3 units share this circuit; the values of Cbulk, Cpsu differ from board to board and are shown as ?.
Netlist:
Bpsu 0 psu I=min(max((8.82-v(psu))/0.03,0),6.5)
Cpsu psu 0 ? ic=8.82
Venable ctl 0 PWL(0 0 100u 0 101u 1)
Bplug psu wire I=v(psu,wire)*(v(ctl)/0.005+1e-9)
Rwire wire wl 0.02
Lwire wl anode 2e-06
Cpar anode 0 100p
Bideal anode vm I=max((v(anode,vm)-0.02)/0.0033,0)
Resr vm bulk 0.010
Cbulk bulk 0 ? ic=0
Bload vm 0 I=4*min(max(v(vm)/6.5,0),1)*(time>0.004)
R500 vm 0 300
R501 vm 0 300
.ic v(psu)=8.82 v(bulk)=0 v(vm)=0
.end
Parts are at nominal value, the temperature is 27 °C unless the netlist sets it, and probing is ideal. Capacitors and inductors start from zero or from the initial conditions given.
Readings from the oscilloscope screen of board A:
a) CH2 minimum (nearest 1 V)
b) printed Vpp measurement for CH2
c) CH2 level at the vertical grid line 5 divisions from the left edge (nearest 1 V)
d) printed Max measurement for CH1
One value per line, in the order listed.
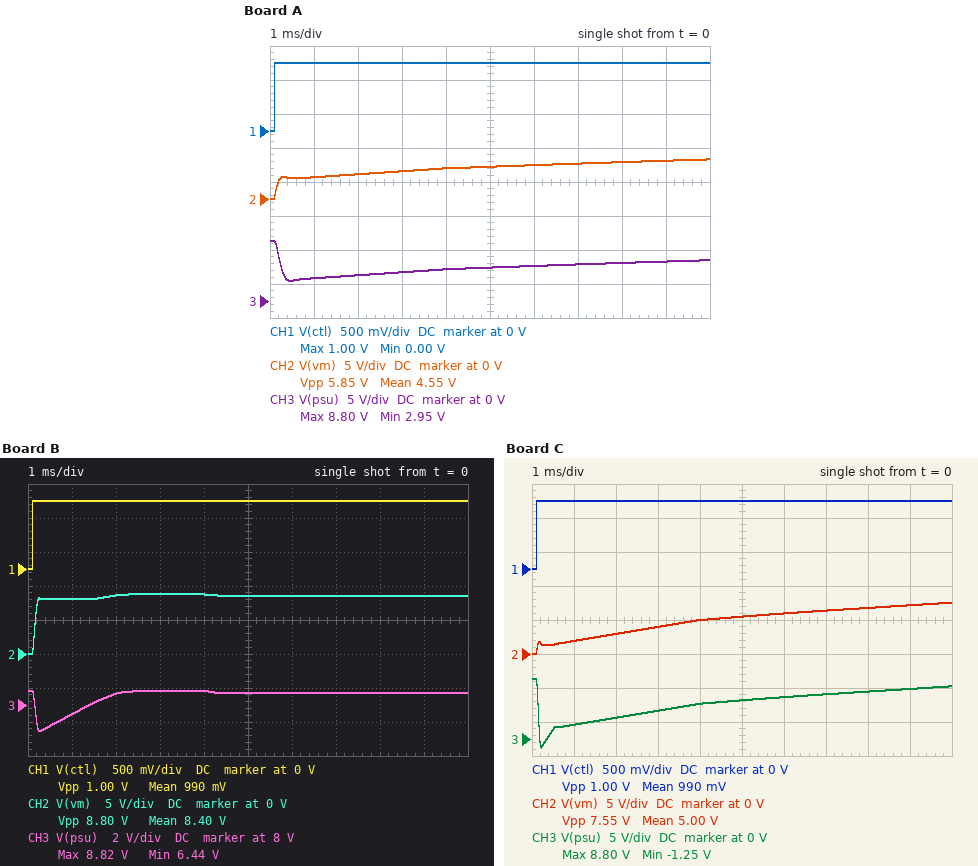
0 V
5.85 V
5 V
1.00 V
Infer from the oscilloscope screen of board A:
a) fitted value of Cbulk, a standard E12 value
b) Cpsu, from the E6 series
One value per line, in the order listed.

10 mF
4.7 mF
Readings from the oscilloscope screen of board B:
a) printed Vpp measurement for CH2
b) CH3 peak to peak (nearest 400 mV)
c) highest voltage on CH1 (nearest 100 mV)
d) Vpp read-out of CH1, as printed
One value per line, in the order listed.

8.80 V
2.4 V
1.0 V
1.00 V
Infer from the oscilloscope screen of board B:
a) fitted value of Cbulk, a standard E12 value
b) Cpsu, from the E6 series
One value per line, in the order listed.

1.5 mF
4.7 mF
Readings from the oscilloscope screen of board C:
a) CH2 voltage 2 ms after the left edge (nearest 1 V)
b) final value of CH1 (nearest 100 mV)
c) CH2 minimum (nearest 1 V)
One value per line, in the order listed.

3 V
1.0 V
0 V
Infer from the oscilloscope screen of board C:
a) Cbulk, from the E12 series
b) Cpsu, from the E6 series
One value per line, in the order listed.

5.6 mF
680 µF
